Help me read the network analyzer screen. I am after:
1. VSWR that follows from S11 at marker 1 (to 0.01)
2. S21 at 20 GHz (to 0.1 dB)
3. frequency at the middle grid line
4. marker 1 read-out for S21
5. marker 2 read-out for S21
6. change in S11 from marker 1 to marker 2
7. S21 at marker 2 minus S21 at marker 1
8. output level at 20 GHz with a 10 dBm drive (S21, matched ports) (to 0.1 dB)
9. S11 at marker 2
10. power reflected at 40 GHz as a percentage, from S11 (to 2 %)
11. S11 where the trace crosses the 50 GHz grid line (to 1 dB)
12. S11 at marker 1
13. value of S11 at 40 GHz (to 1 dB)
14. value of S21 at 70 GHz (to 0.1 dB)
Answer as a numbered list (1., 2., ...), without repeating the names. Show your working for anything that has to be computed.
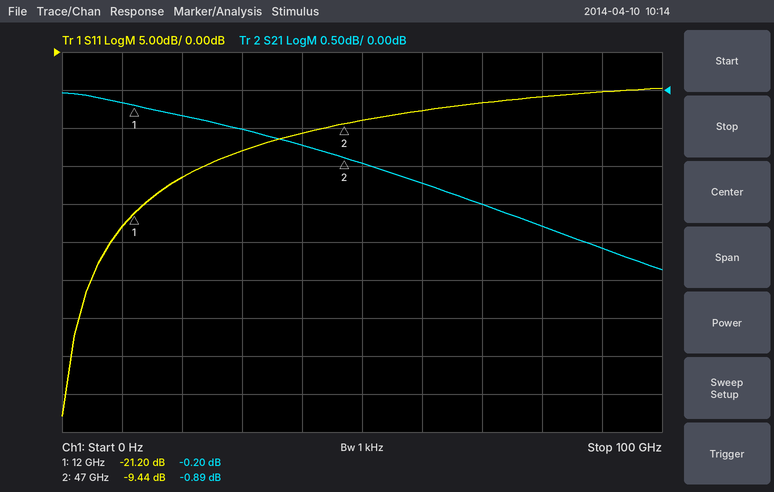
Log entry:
1. (1 + 0.0871)/(1 − 0.0871) ≈ 1.19
2. -0.3 dB
3. 50 GHz
4. -0.20 dB
5. -0.89 dB
6. -9.44 − (-21.2) = 11.76 dB
7. -0.89 − (-0.2) = -0.69 dB
8. 10 dBm + (-0.3 dB) = 9.7 dBm
9. -9.44 dB
10. 10^(-11/10) ≈ 8 %
11. -9 dB
12. -21.20 dB
13. -11 dB
14. -1.5 dB
